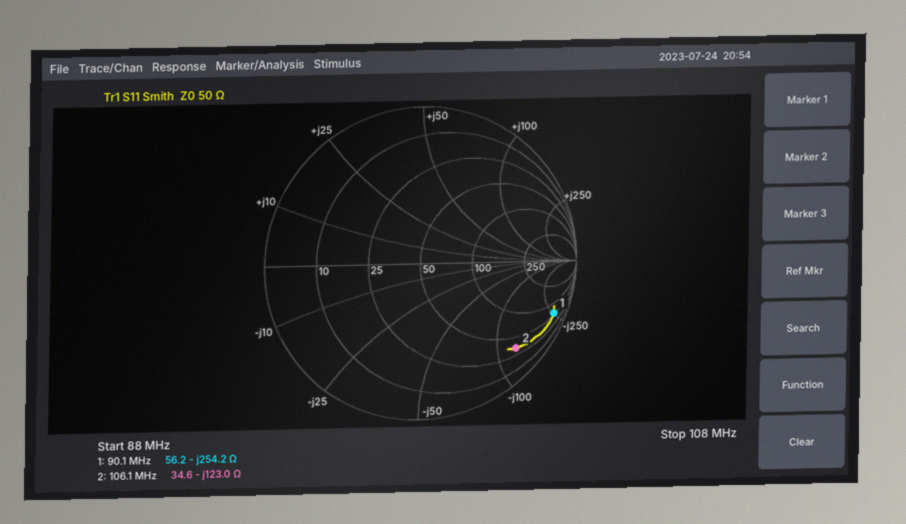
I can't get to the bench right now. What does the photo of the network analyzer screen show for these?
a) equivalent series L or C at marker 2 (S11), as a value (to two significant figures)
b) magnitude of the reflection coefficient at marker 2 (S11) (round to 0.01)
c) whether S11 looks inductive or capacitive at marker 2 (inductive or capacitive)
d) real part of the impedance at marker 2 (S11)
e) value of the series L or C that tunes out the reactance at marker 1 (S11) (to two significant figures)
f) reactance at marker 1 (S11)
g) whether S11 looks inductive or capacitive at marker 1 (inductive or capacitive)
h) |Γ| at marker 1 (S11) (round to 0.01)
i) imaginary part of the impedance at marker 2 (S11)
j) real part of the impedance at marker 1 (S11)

12 pF
0.83
capacitive
34.6 Ω
450 nH
-254.2 Ω
capacitive
0.92
-123.0 Ω
56.2 Ω
